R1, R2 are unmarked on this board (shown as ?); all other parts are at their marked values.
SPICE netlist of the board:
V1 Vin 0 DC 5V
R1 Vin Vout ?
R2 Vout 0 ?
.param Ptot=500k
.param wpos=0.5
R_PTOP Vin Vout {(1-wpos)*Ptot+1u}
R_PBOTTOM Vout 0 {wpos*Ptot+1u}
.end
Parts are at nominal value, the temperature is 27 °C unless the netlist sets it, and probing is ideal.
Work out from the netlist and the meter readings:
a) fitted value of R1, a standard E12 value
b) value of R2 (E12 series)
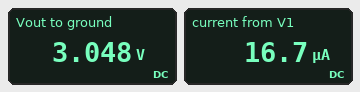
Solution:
220 kΩ
680 kΩ
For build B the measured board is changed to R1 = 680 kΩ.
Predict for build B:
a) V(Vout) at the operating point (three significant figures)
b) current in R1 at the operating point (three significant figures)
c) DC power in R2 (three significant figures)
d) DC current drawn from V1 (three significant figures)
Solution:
2.50 V
3.68 µA
9.19 µW
13.7 µA
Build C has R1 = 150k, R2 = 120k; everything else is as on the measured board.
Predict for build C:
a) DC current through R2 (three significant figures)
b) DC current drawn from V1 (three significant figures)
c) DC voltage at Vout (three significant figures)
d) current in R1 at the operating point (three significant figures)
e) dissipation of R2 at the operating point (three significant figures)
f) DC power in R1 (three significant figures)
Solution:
19.3 µA
28.6 µA
2.32 V
17.9 µA
44.8 µW
47.9 µW
